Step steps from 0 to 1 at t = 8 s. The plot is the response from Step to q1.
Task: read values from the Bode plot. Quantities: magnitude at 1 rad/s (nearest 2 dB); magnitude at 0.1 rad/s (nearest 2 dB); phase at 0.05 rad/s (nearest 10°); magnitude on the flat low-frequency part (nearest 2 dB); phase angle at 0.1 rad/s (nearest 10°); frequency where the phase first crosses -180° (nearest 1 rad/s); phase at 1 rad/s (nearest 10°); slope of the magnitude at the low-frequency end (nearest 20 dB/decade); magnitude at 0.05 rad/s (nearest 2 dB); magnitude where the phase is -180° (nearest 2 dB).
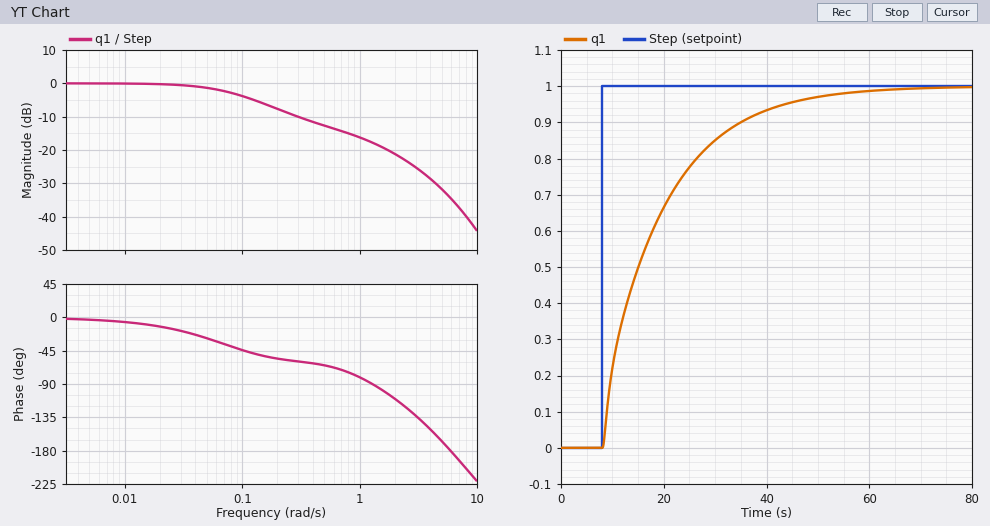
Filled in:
-16 dB
-4 dB
-30°
0 dB
-40°
6 rad/s
-80°
0 dB/decade
-2 dB
-34 dB
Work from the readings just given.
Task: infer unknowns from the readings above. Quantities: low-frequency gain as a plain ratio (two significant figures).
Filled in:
1.0
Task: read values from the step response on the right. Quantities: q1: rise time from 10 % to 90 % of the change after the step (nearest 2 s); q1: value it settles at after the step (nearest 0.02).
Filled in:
26 s
1.00
